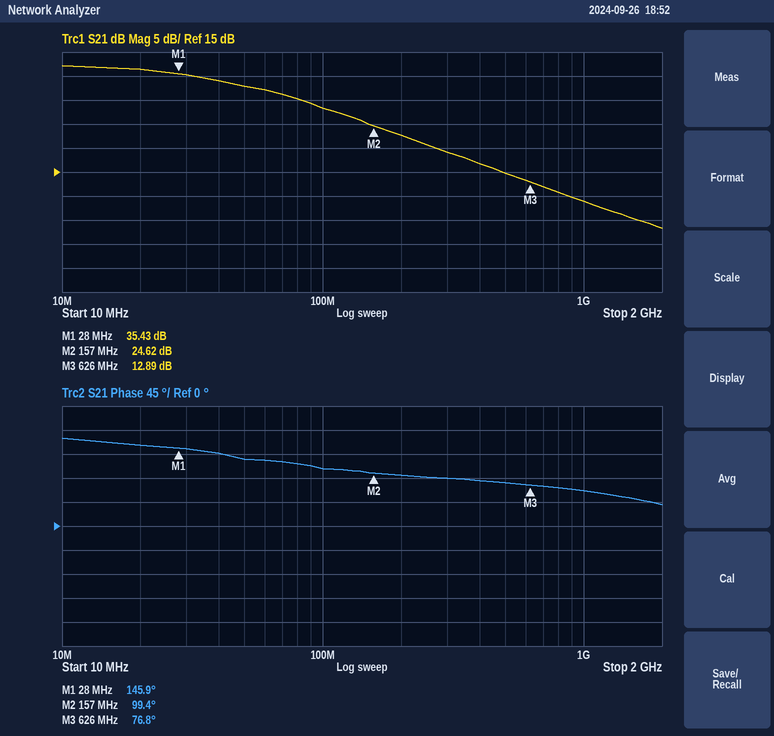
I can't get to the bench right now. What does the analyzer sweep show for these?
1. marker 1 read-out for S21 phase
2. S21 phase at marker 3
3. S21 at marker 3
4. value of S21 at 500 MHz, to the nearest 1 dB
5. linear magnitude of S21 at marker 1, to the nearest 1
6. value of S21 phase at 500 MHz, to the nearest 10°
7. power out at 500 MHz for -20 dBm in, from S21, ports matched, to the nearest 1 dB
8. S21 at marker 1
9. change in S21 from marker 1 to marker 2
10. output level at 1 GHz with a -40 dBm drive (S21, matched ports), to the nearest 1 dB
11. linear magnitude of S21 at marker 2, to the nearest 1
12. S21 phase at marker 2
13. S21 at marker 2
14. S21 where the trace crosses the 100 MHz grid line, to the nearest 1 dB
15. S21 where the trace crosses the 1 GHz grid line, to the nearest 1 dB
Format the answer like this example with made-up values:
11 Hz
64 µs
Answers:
145.9°
76.8°
12.89 dB
15 dB
59
80°
-5 dBm
35.43 dB
-10.81 dB
-31 dBm
17
99.4°
24.62 dB
28 dB
9 dB
